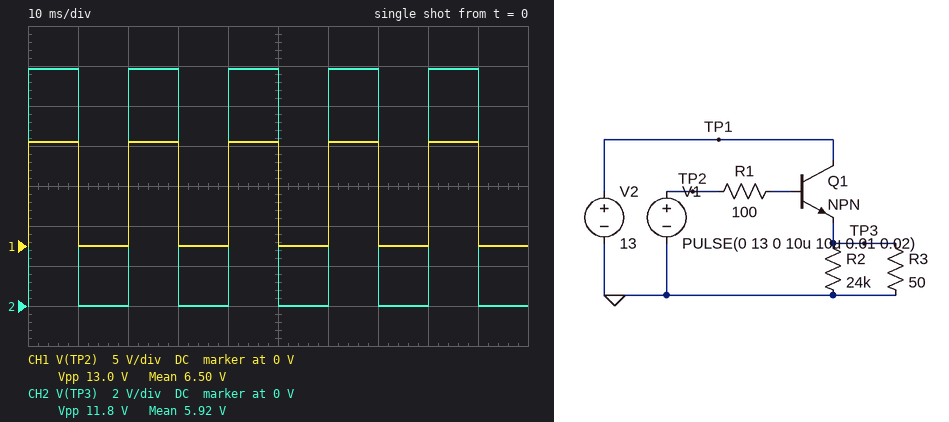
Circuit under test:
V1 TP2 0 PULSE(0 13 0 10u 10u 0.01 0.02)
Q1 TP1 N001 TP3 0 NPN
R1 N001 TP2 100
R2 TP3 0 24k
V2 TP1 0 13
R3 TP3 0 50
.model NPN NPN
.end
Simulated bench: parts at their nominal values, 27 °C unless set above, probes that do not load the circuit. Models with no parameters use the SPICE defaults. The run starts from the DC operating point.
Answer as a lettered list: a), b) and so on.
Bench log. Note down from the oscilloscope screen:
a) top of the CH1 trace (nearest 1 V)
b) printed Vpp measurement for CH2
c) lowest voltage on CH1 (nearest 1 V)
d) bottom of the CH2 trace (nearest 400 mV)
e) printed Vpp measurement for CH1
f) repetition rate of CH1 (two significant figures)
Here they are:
a) 13 V
b) 11.8 V
c) 0 V
d) 0 V
e) 13.0 V
f) 50 Hz
